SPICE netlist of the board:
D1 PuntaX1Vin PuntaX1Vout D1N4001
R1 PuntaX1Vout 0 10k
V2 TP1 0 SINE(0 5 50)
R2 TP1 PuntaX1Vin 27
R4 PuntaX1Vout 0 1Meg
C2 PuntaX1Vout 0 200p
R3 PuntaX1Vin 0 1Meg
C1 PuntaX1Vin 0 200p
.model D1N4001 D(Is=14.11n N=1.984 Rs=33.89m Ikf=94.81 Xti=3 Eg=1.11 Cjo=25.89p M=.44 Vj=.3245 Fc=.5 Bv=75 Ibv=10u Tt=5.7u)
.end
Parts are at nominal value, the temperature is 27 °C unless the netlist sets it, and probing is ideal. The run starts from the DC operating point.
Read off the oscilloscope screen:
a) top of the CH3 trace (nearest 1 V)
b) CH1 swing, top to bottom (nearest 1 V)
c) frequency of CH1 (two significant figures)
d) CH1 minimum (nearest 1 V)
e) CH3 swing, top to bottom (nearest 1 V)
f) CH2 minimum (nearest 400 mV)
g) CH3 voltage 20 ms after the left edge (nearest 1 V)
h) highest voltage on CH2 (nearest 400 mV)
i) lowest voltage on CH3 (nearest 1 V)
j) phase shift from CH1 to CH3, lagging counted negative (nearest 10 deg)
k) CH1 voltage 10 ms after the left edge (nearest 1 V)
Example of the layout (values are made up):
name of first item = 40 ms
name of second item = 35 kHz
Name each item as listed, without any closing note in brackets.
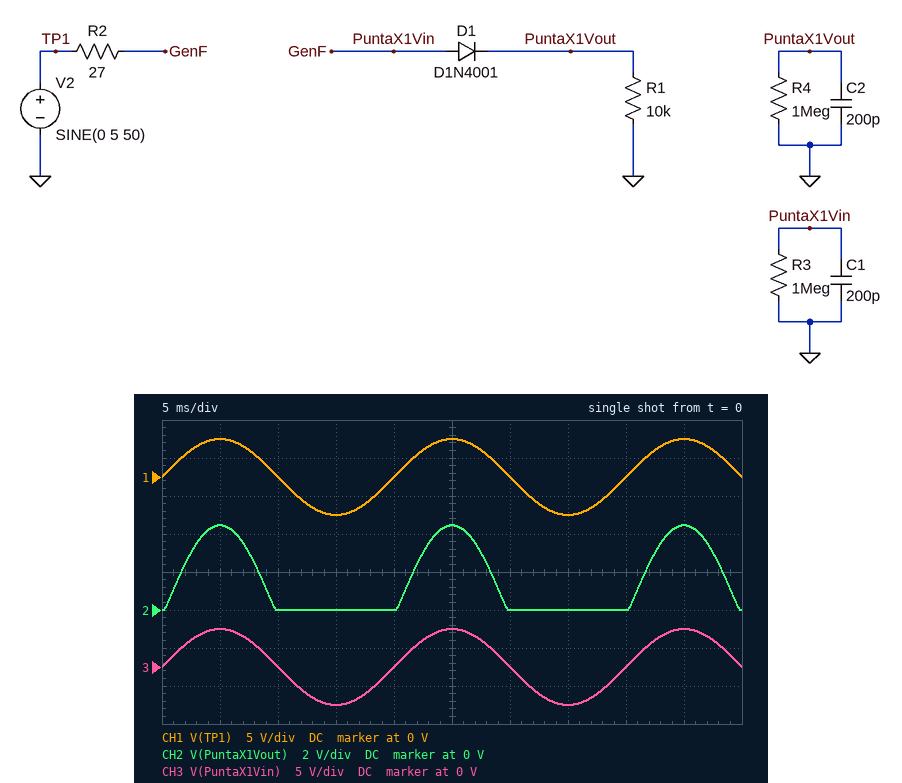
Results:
top of the CH3 trace = 5 V
CH1 swing, top to bottom = 10 V
frequency of CH1 = 50 Hz
CH1 minimum = -5 V
CH3 swing, top to bottom = 10 V
CH2 minimum = 0 V
CH3 voltage 20 ms after the left edge = 0 V
highest voltage on CH2 = 4.4 V
lowest voltage on CH3 = -5 V
phase shift from CH1 to CH3, lagging counted negative = 0 deg
CH1 voltage 10 ms after the left edge = 0 V
